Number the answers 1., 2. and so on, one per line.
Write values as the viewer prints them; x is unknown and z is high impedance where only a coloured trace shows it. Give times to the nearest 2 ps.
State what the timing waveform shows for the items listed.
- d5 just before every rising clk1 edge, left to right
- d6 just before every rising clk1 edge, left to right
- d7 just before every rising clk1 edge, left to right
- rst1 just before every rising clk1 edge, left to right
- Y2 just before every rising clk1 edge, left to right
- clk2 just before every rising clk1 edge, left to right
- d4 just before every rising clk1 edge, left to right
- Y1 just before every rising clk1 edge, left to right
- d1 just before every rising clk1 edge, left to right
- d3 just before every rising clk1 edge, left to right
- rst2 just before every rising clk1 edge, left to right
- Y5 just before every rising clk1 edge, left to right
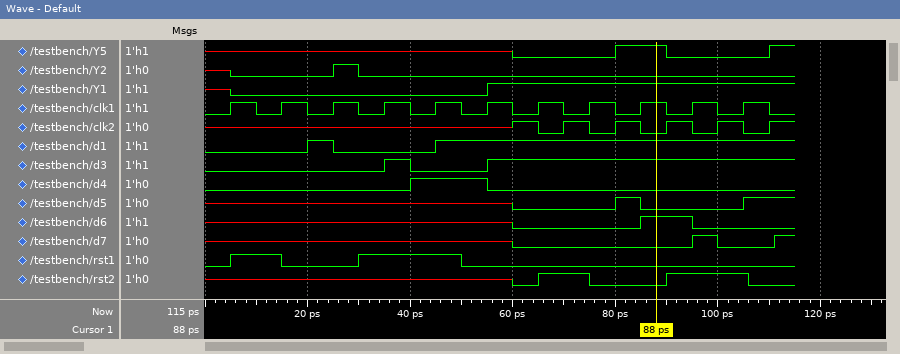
1. x x x x x x 0 0 1 0 0
2. x x x x x x 0 0 0 1 0
3. x x x x x x 0 0 0 0 0
4. 0 1 0 1 1 0 0 0 0 0 0
5. x 0 0 0 0 0 0 0 0 0 0
6. x x x x x x 1 1 1 1 1
7. 0 0 0 0 1 1 0 0 0 0 0
8. x 0 0 0 0 0 1 1 1 1 1
9. 0 0 1 0 0 1 1 1 1 1 1
10. 0 0 0 0 0 0 1 1 1 1 1
11. x x x x x x 0 1 0 1 1
12. x x x x x x 0 0 1 0 0
